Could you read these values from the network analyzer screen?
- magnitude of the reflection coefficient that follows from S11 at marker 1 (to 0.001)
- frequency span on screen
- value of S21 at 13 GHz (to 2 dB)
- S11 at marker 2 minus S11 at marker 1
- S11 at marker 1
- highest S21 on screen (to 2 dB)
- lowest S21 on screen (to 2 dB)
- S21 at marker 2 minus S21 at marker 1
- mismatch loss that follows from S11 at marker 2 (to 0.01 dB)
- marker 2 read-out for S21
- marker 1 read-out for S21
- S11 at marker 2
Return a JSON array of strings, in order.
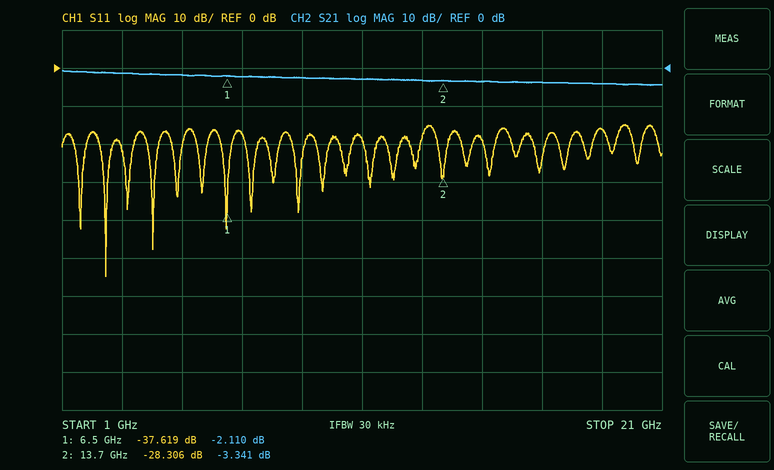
["0.013", "20 GHz", "-4 dB", "9.313 dB", "-37.619 dB", "0 dB", "-4 dB", "-1.231 dB", "0.01 dB", "-3.341 dB", "-2.110 dB", "-28.306 dB"]
